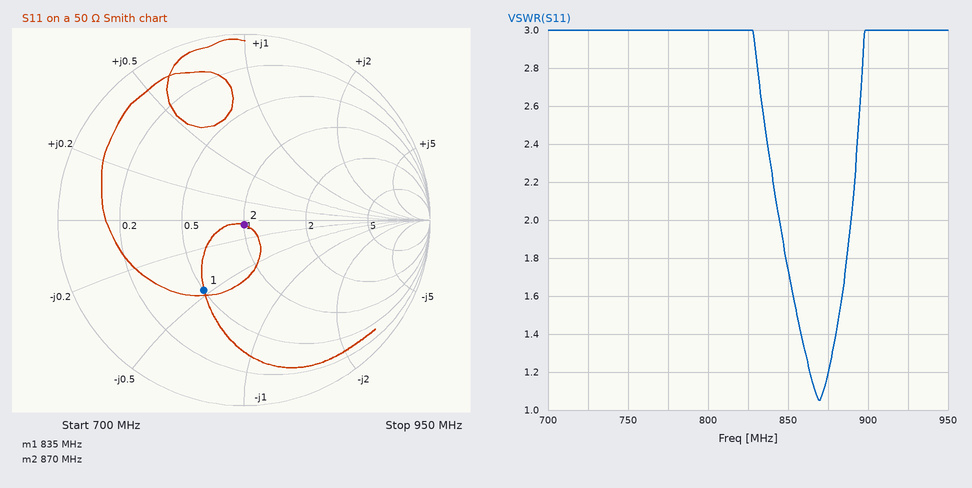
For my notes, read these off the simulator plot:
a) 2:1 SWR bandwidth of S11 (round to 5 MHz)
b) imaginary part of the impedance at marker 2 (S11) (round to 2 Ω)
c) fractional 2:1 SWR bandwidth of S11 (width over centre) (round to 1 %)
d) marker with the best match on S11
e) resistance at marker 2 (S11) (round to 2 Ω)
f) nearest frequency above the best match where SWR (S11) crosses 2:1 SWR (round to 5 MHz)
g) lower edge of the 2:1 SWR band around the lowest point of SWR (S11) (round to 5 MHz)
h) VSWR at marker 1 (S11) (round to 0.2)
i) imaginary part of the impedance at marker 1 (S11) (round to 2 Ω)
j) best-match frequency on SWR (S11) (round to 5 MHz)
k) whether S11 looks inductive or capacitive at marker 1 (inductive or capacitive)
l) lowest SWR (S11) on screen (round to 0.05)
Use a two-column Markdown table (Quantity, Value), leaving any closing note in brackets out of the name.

| Quantity | Value |
|---|---|
| 2:1 SWR bandwidth of S11 | 45 MHz |
| imaginary part of the impedance at marker 2 (S11) | -2 Ω |
| fractional 2:1 SWR bandwidth of S11 (width over centre) | 5 % |
| marker with the best match on S11 | marker 2 |
| resistance at marker 2 (S11) | 50 Ω |
| nearest frequency above the best match where SWR (S11) crosses 2:1 SWR | 890 MHz |
| lower edge of the 2:1 SWR band around the lowest point of SWR (S11) | 845 MHz |
| VSWR at marker 1 (S11) | 2.6 |
| imaginary part of the impedance at marker 1 (S11) | -24 Ω |
| best-match frequency on SWR (S11) | 870 MHz |
| whether S11 looks inductive or capacitive at marker 1 | capacitive |
| lowest SWR (S11) on screen | 1.05 |
